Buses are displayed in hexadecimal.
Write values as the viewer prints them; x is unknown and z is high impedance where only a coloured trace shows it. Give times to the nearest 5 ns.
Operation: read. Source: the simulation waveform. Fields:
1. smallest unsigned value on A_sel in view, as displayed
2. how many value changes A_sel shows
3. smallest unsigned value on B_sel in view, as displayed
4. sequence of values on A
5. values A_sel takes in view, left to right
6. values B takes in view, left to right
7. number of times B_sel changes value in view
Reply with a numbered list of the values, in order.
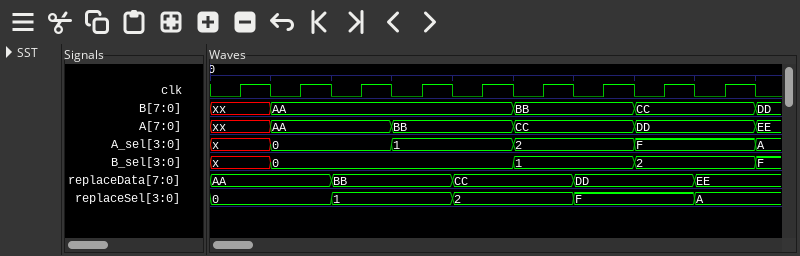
1. 0
2. 5
3. 0
4. xx, AA, BB, CC, DD, EE
5. x, 0, 1, 2, F, A
6. xx, AA, BB, CC, DD
7. 4
